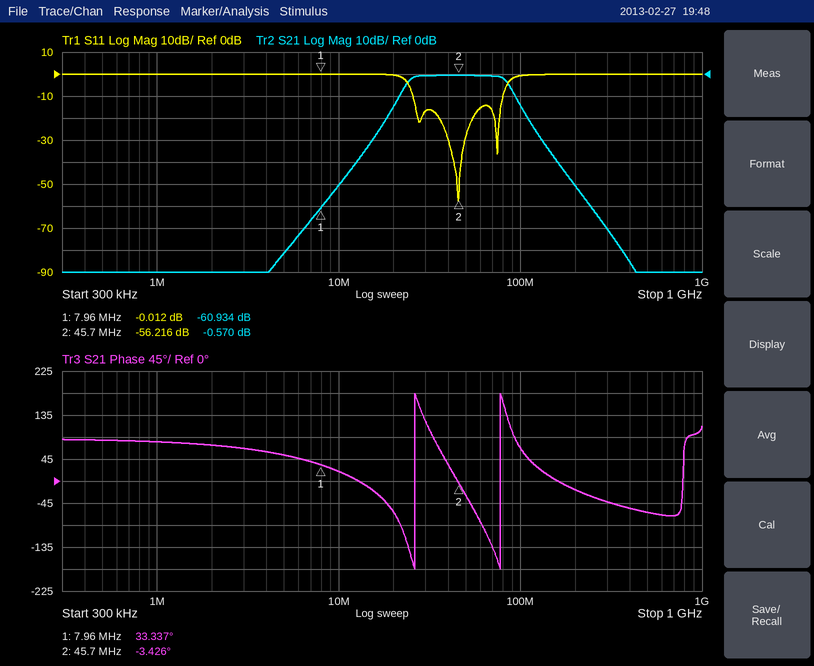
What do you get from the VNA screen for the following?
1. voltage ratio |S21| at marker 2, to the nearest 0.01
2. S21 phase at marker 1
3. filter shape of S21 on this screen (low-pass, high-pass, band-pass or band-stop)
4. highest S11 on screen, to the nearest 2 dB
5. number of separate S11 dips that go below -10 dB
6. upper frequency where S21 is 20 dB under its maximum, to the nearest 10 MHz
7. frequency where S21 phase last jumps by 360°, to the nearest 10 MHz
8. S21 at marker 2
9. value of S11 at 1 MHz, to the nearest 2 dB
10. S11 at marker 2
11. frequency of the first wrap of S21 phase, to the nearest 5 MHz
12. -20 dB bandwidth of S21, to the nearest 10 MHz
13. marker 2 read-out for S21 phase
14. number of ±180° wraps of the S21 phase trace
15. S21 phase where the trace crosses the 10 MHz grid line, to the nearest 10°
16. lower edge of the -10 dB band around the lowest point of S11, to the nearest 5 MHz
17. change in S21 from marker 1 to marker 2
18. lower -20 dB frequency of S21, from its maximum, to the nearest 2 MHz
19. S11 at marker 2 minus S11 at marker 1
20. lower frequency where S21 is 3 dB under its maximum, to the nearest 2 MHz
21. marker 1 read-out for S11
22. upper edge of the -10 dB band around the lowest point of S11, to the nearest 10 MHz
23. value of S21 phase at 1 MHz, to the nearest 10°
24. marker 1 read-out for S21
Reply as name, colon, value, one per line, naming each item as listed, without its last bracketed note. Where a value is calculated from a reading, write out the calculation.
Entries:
voltage ratio |S21| at marker 2, to the nearest 0.01: 10^(-0.57/20) ≈ 0.94
S21 phase at marker 1: 33.337°
filter shape of S21 on this screen: band-pass
highest S11 on screen, to the nearest 2 dB: 0 dB
number of separate S11 dips that go below -10 dB: 3
upper frequency where S21 is 20 dB under its maximum, to the nearest 10 MHz: 110 MHz
frequency where S21 phase last jumps by 360°, to the nearest 10 MHz: 80 MHz
S21 at marker 2: -0.570 dB
value of S11 at 1 MHz, to the nearest 2 dB: 0 dB
S11 at marker 2: -56.216 dB
frequency of the first wrap of S21 phase, to the nearest 5 MHz: 25 MHz
-20 dB bandwidth of S21, to the nearest 10 MHz: 110 MHz − 18 MHz = 92 MHz
marker 2 read-out for S21 phase: -3.426°
number of ±180° wraps of the S21 phase trace: 2
S21 phase where the trace crosses the 10 MHz grid line, to the nearest 10°: 20°
lower edge of the -10 dB band around the lowest point of S11, to the nearest 5 MHz: 25 MHz
change in S21 from marker 1 to marker 2: -0.57 − (-60.934) = 60.364 dB
lower -20 dB frequency of S21, from its maximum, to the nearest 2 MHz: 18 MHz
S11 at marker 2 minus S11 at marker 1: -56.216 − (-0.012) = -56.204 dB
lower frequency where S21 is 3 dB under its maximum, to the nearest 2 MHz: 24 MHz
marker 1 read-out for S11: -0.012 dB
upper edge of the -10 dB band around the lowest point of S11, to the nearest 10 MHz: 80 MHz
value of S21 phase at 1 MHz, to the nearest 10°: 80°
marker 1 read-out for S21: -60.934 dB
